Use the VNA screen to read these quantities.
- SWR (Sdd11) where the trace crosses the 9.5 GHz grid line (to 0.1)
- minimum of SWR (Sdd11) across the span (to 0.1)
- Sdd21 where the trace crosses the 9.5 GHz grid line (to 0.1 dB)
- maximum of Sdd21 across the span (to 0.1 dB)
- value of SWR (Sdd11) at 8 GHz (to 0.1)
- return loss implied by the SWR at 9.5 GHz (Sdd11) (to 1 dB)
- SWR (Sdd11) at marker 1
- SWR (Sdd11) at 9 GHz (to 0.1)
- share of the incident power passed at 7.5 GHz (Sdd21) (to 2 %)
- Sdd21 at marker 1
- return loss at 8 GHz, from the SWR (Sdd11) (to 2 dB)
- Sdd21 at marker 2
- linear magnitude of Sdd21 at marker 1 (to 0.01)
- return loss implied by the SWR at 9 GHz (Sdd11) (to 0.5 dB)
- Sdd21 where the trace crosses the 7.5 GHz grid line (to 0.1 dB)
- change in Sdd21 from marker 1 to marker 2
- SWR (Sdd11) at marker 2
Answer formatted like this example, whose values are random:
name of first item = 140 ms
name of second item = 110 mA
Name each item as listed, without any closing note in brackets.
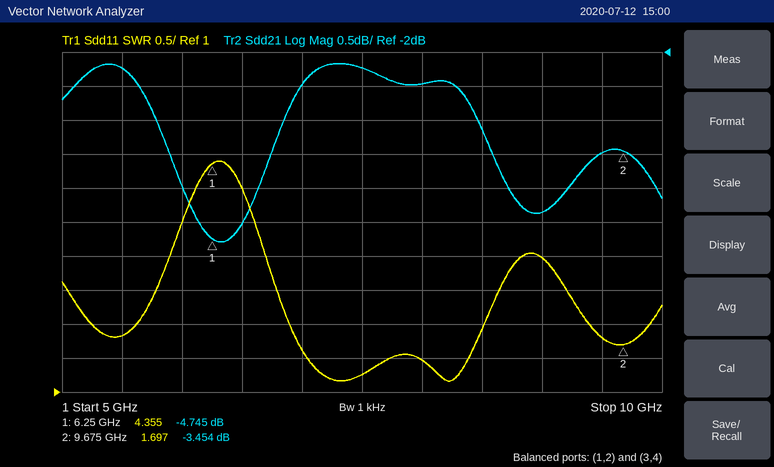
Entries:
SWR (Sdd11) where the trace crosses the 9.5 GHz grid line = 1.8
minimum of SWR (Sdd11) across the span = 1.2
Sdd21 where the trace crosses the 9.5 GHz grid line = -3.5 dB
maximum of Sdd21 across the span = -2.2 dB
value of SWR (Sdd11) at 8 GHz = 1.5
return loss implied by the SWR at 9.5 GHz (Sdd11) = 11 dB
SWR (Sdd11) at marker 1 = 4.355
SWR (Sdd11) at 9 GHz = 3.0
share of the incident power passed at 7.5 GHz (Sdd21) = 60 %
Sdd21 at marker 1 = -4.745 dB
return loss at 8 GHz, from the SWR (Sdd11) = 14 dB
Sdd21 at marker 2 = -3.454 dB
linear magnitude of Sdd21 at marker 1 = 0.58
return loss implied by the SWR at 9 GHz (Sdd11) = 6.0 dB
Sdd21 where the trace crosses the 7.5 GHz grid line = -2.2 dB
change in Sdd21 from marker 1 to marker 2 = 1.291 dB
SWR (Sdd11) at marker 2 = 1.697
